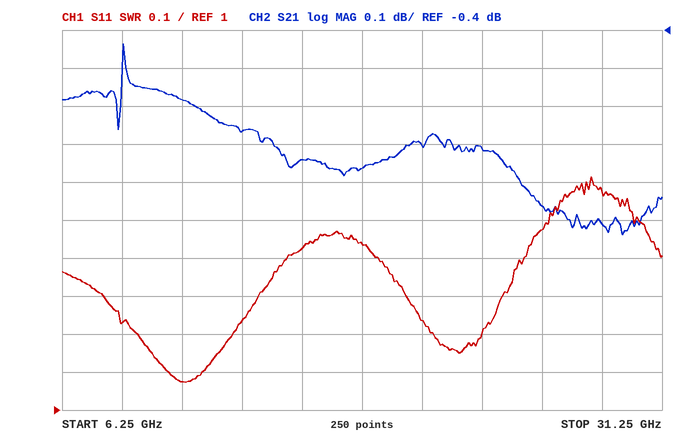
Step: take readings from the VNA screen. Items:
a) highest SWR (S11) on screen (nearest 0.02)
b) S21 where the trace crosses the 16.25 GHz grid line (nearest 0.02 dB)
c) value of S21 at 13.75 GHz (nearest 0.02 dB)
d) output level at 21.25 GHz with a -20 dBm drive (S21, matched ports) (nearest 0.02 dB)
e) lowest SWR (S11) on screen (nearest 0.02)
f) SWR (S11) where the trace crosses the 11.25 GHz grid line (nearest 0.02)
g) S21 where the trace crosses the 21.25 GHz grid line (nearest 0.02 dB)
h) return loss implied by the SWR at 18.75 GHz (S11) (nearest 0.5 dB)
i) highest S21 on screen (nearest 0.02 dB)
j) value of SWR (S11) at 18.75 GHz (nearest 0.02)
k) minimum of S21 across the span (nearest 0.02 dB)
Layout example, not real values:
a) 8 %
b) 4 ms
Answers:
a) 1.62
b) -0.74 dB
c) -0.66 dB
d) -20.70 dBm
e) 1.08
f) 1.08
g) -0.70 dB
h) 15.0 dB
i) -0.44 dB
j) 1.44
k) -0.94 dB
